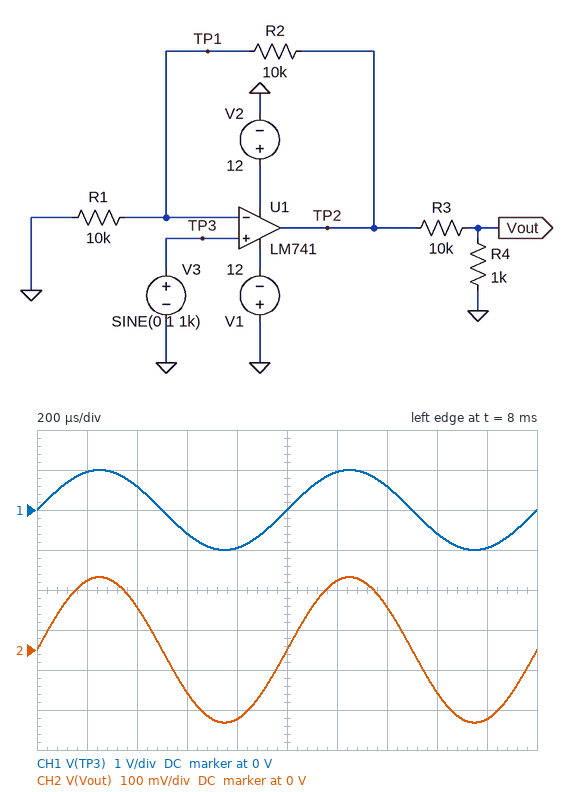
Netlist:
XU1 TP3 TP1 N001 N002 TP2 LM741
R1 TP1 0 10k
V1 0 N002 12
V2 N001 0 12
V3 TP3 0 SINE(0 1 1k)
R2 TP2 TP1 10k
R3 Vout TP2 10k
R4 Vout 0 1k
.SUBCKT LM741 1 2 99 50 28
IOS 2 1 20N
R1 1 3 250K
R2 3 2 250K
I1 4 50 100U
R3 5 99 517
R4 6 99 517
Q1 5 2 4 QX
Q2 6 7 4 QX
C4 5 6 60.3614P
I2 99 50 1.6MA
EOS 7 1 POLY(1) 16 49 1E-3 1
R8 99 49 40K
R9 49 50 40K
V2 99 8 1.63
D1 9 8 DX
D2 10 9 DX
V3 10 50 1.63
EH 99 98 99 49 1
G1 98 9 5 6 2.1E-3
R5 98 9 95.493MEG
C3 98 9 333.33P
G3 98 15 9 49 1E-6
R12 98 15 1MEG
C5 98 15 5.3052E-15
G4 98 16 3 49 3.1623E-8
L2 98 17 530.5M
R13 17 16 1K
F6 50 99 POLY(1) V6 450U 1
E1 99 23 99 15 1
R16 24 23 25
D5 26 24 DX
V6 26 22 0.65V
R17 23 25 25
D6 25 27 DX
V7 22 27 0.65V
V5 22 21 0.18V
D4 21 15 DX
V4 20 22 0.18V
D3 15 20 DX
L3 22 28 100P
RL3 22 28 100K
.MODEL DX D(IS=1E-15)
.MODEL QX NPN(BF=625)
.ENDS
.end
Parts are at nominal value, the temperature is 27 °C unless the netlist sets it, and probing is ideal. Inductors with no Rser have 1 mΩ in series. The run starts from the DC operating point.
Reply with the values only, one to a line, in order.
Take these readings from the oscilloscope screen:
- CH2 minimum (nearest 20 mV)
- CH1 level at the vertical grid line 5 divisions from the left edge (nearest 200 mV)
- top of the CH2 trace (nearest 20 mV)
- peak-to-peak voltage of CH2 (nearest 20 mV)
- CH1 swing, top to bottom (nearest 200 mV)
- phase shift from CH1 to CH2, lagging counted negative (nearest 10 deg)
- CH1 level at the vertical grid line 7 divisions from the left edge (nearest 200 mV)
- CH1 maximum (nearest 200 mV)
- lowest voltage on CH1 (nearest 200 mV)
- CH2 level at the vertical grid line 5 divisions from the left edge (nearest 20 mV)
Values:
-180 mV
0 V
180 mV
360 mV
2.0 V
0 deg
600 mV
1.0 V
-1.0 V
0 V
